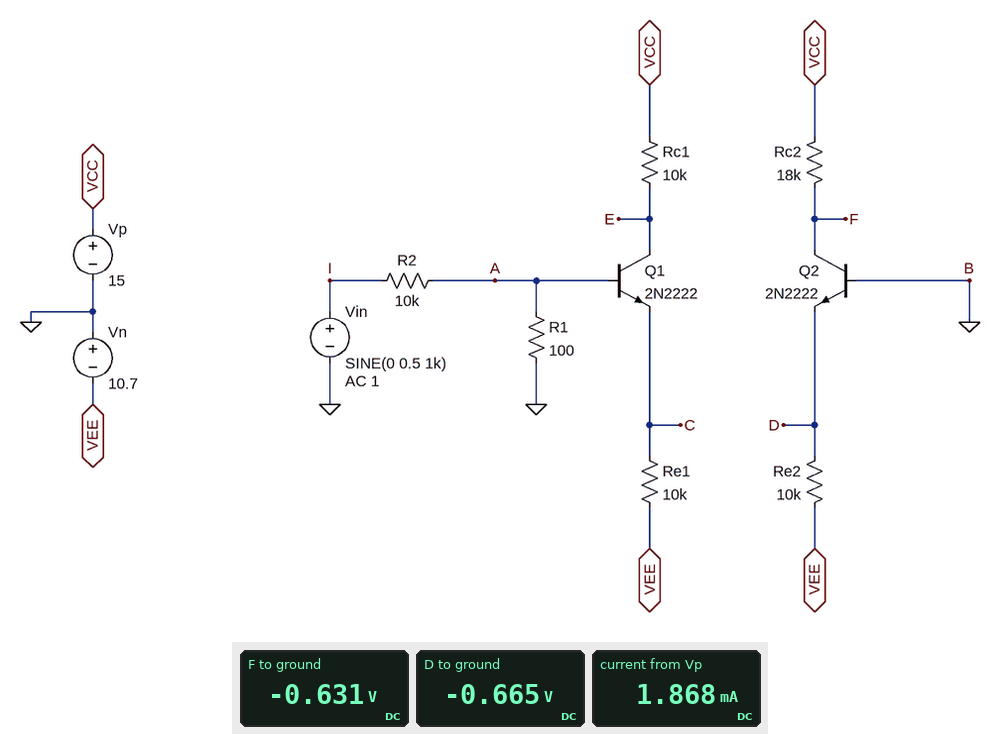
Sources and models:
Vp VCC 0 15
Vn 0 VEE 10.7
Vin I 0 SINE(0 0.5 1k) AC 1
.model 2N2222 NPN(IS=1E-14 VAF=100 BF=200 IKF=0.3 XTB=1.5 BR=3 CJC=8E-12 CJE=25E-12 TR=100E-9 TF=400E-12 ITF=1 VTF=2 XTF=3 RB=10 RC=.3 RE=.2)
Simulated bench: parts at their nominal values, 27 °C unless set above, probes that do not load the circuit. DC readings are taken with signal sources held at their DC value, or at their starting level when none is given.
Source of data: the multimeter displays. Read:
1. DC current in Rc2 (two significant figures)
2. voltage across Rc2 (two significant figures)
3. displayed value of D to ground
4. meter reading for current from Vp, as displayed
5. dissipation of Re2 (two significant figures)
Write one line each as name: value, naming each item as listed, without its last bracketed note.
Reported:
DC current in Rc2: 870 µA
voltage across Rc2: 16 V
displayed value of D to ground: -0.665 V
meter reading for current from Vp, as displayed: 1.868 mA
dissipation of Re2: 10 mW
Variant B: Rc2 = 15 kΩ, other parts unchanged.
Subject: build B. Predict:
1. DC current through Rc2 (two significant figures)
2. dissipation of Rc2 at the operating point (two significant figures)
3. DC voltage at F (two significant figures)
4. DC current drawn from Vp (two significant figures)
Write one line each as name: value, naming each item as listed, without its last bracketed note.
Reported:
DC current through Rc2: 1.0 mA
dissipation of Rc2 at the operating point: 15 mW
DC voltage at F: 8.4 mV
DC current drawn from Vp: 2.0 mA
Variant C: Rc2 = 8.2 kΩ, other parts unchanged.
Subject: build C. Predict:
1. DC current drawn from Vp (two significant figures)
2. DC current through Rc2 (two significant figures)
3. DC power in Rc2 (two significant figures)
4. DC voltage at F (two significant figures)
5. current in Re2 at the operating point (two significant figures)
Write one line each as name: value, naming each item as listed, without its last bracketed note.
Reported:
DC current drawn from Vp: 2.0 mA
DC current through Rc2: 1.0 mA
DC power in Rc2: 8.2 mW
DC voltage at F: 6.8 V
current in Re2 at the operating point: 1.0 mA
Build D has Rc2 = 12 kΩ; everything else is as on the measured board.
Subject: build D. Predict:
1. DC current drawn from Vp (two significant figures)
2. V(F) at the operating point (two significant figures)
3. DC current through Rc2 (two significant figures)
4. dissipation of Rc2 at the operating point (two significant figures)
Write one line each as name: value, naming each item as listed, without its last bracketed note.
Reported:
DC current drawn from Vp: 2.0 mA
V(F) at the operating point: 3.0 V
DC current through Rc2: 1.0 mA
dissipation of Rc2 at the operating point: 12 mW
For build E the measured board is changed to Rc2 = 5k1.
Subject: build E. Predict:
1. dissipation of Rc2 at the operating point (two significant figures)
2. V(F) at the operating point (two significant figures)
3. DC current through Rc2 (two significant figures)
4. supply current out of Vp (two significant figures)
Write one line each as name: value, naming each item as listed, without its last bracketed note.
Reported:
dissipation of Rc2 at the operating point: 5.1 mW
V(F) at the operating point: 9.9 V
DC current through Rc2: 1.0 mA
supply current out of Vp: 2.0 mA
